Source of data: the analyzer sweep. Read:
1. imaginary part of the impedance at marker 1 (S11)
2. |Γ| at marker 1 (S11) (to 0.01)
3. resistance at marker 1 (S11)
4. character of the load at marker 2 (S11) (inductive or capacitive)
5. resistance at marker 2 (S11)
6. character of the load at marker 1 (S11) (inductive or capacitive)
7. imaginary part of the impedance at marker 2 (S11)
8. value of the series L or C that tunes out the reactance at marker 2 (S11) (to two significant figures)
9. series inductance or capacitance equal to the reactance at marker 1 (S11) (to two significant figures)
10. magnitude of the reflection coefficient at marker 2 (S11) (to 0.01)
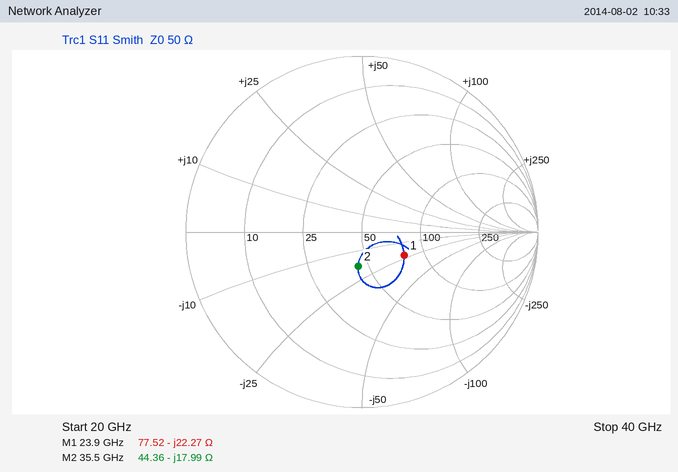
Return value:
-22.27 Ω
0.27
77.52 Ω
capacitive
44.36 Ω
capacitive
-17.99 Ω
81 pH
300 fF
0.20
